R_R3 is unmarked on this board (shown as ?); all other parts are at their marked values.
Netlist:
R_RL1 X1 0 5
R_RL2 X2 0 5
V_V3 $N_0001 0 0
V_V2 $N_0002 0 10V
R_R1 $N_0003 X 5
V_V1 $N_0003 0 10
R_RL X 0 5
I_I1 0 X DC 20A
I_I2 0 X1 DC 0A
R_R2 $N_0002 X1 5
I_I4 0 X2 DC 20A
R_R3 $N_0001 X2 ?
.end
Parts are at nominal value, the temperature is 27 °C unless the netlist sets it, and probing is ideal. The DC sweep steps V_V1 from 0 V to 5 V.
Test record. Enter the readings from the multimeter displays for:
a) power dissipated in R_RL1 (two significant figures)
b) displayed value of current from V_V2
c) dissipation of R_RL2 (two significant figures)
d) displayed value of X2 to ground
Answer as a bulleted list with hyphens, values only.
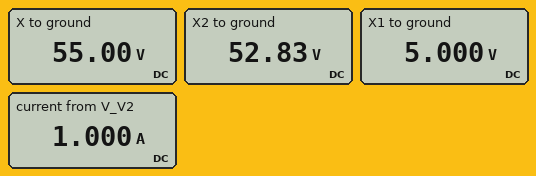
- 5.0 W
- 1.000 A
- 560 W
- 52.83 V
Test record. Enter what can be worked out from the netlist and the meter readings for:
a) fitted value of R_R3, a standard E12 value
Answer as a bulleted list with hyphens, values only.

- 5.6 Ω
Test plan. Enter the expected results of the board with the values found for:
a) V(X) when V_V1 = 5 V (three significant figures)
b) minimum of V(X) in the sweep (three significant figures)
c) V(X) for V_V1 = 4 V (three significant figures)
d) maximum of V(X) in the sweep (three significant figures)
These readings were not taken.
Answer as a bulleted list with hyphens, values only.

- 52.5 V
- 50.0 V
- 52.0 V
- 52.5 V
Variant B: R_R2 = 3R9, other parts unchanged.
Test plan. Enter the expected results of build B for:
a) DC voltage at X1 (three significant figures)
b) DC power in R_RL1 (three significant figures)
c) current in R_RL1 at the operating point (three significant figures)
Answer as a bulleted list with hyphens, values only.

- 5.62 V
- 6.31 W
- 1.12 A
